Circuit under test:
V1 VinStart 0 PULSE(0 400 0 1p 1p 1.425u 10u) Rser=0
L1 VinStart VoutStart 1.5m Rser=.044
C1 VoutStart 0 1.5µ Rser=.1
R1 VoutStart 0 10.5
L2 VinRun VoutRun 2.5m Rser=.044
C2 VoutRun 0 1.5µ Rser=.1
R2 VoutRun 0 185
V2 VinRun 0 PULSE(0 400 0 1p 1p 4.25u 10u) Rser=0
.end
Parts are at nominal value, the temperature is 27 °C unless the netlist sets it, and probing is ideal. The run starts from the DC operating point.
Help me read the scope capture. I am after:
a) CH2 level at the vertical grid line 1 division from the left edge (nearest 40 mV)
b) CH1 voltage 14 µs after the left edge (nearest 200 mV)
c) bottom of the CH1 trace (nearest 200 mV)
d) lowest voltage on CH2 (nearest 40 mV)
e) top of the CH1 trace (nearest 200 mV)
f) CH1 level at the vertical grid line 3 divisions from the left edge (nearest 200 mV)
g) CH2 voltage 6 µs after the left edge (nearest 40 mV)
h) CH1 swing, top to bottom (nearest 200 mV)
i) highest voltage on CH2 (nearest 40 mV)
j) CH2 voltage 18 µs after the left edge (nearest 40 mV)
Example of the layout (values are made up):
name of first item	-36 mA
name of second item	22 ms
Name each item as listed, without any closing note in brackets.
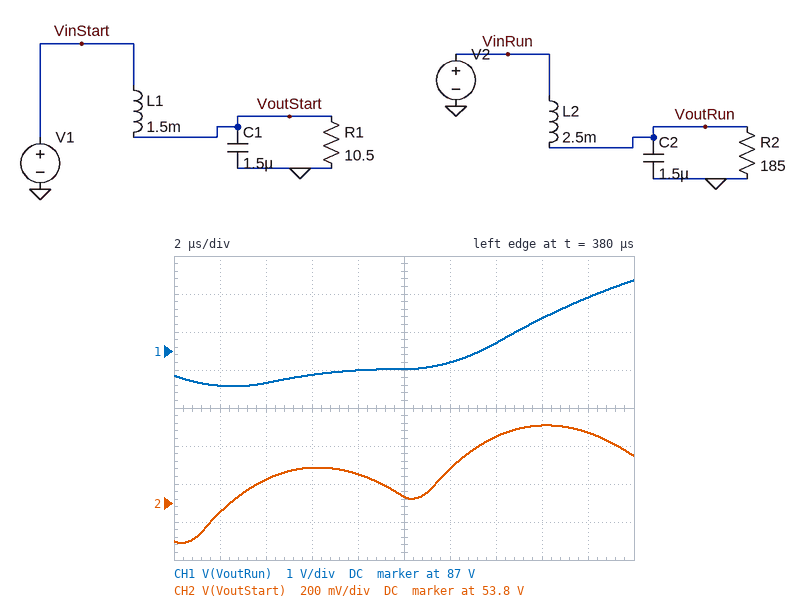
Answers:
CH2 level at the vertical grid line 1 division from the left edge	53.76 V
CH1 voltage 14 µs after the left edge	87.2 V
bottom of the CH1 trace	86.0 V
lowest voltage on CH2	53.60 V
top of the CH1 trace	88.8 V
CH1 level at the vertical grid line 3 divisions from the left edge	86.4 V
CH2 voltage 6 µs after the left edge	54.00 V
CH1 swing, top to bottom	2.8 V
highest voltage on CH2	54.20 V
CH2 voltage 18 µs after the left edge	54.16 V
